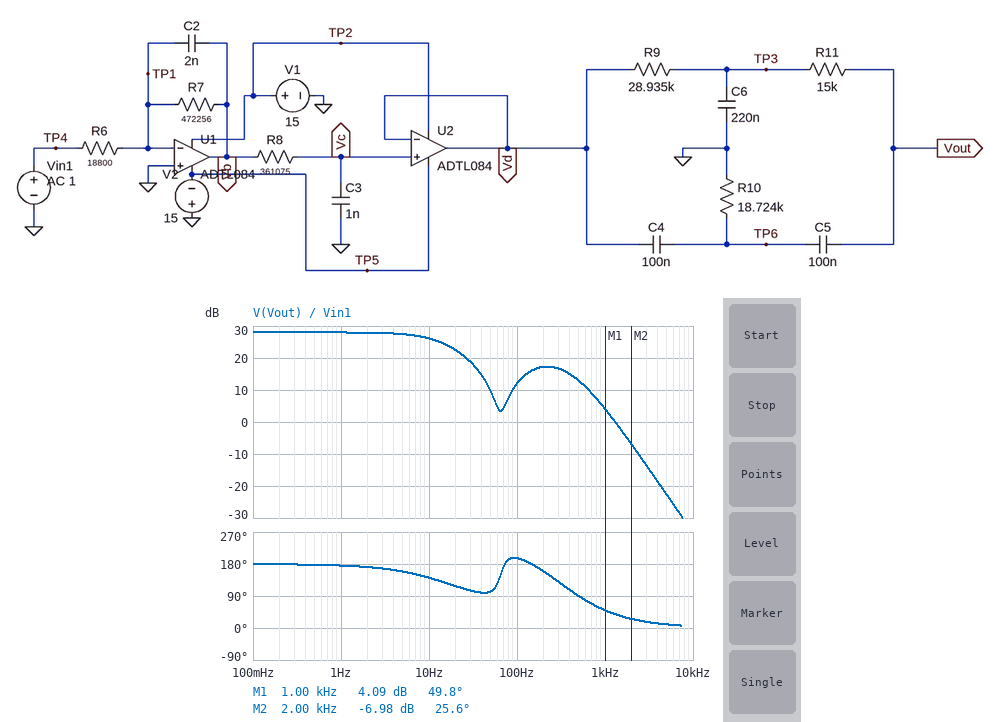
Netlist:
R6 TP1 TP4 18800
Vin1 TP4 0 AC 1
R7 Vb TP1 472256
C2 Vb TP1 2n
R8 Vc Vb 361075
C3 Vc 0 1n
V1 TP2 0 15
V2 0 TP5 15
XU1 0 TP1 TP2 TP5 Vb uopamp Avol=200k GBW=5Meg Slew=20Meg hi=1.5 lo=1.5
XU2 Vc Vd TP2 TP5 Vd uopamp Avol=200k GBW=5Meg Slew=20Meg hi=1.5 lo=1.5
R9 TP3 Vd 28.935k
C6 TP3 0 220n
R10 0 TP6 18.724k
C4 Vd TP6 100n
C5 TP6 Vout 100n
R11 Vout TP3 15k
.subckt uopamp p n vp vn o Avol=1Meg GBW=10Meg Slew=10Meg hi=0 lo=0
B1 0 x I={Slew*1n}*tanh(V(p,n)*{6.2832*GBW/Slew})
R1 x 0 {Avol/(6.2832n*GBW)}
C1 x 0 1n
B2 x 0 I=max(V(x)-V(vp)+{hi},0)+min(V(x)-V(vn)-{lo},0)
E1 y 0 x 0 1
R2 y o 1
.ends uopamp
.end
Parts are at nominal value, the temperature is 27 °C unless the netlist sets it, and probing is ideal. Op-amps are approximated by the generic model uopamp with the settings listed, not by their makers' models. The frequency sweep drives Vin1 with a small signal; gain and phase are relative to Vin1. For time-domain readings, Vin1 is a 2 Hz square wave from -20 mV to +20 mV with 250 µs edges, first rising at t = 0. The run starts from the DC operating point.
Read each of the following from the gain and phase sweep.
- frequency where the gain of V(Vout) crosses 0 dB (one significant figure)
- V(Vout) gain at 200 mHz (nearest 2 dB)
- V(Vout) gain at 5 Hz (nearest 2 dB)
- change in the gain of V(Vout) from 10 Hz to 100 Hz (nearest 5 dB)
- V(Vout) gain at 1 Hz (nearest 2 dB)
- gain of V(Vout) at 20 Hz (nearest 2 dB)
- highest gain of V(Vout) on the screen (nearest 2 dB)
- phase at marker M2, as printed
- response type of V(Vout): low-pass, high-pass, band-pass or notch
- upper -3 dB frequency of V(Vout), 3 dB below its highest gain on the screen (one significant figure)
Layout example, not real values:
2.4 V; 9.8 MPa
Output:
1 kHz; 28 dB; 28 dB; -15 dB; 28 dB; 22 dB; 28 dB; 25.6 deg; low-pass; 10 Hz
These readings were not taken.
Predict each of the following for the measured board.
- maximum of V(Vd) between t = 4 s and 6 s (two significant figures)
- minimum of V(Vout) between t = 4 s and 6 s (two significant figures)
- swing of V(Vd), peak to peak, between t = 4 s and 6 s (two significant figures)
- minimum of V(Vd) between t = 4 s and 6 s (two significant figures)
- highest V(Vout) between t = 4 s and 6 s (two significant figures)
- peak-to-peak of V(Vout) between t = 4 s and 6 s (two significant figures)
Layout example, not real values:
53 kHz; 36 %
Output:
500 mV; -500 mV; 1.0 V; -500 mV; 500 mV; 1.0 V
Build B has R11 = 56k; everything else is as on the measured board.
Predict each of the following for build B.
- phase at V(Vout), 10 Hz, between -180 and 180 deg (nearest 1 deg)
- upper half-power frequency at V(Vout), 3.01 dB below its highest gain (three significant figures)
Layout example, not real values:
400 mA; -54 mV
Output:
130 deg; 10.1 Hz
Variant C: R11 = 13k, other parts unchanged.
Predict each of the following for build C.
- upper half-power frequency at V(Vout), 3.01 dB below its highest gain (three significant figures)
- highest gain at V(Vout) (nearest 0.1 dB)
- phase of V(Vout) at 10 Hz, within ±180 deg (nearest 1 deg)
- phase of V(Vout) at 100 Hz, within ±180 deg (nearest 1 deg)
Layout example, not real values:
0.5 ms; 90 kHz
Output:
13.5 Hz; 28.0 dB; 142 deg; -169 deg
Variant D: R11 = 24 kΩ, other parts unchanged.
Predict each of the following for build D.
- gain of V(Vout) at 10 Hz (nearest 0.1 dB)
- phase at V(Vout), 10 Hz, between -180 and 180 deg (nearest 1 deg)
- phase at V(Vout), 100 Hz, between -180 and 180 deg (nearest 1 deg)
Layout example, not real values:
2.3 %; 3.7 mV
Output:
25.9 dB; 139 deg; -157 deg
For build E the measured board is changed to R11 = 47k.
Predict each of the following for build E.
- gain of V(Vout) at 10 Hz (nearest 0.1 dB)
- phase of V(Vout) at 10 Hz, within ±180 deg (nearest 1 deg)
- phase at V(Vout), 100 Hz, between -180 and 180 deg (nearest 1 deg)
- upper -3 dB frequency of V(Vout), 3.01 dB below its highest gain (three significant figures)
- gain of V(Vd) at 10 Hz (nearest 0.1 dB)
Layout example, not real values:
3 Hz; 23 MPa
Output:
25.3 dB; 132 deg; -161 deg; 10.7 Hz; 28.0 dB
